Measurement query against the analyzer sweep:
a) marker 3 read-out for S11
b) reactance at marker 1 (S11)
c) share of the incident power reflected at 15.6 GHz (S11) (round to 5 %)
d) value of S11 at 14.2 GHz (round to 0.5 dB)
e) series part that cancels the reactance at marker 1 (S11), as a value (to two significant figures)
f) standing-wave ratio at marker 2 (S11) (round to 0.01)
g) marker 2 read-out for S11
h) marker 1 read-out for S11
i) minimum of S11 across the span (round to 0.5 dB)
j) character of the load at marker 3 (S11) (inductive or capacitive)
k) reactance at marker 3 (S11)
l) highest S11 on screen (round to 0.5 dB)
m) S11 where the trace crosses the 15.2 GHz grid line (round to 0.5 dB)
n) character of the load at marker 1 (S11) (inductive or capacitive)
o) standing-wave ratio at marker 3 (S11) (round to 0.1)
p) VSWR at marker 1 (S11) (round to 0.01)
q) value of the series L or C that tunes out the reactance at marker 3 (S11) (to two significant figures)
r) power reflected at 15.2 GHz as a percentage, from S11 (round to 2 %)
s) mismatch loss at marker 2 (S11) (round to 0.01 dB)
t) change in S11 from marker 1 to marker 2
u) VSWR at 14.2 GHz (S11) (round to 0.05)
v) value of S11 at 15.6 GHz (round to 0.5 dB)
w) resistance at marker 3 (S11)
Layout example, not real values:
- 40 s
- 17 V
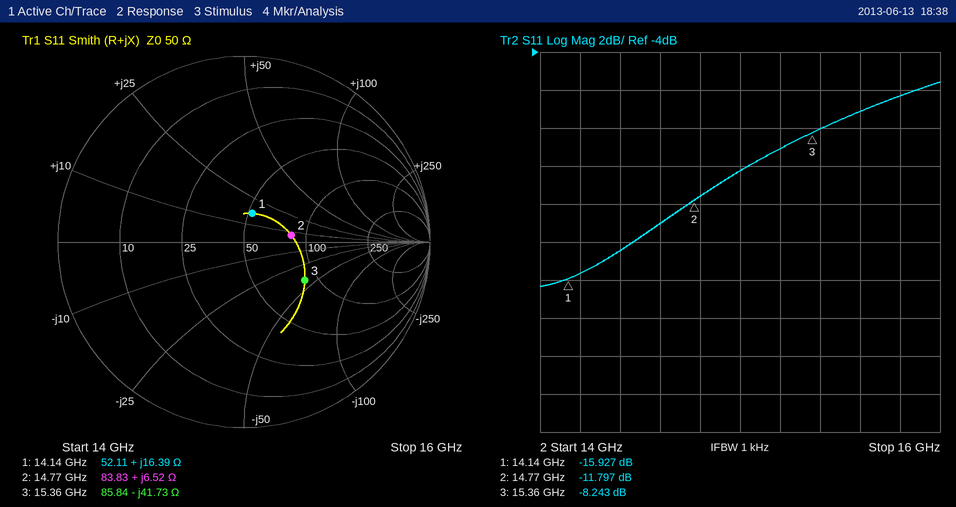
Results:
- -8.243 dB
- +16.39 Ω
- 20 %
- -15.5 dB
- 690 fF
- 1.69
- -11.797 dB
- -15.927 dB
- -16.5 dB
- capacitive
- -41.73 Ω
- -5.5 dB
- -9.0 dB
- inductive
- 2.3
- 1.38
- 430 pH
- 12 %
- 0.30 dB
- 4.130 dB
- 1.40
- -7.0 dB
- 85.84 Ω
